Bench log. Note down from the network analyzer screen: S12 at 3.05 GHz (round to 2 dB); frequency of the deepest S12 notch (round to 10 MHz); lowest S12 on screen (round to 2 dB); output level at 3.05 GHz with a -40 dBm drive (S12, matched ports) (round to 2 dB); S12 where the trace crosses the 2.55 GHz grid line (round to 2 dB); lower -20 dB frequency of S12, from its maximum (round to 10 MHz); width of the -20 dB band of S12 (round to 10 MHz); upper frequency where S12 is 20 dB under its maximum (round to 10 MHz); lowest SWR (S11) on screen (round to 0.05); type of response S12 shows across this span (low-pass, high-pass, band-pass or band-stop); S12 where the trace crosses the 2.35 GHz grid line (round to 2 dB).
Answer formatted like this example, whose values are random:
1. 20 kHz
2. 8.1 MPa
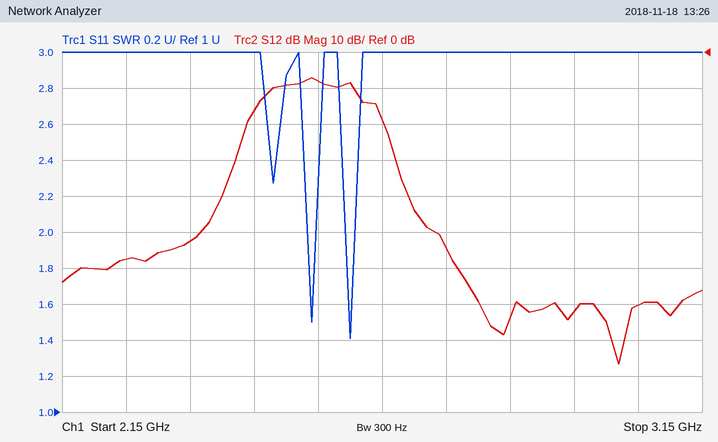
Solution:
1. -70 dB
2. 3.02 GHz
3. -86 dB
4. -110 dBm
5. -8 dB
6. 2.43 GHz
7. 240 MHz
8. 2.67 GHz
9. 1.40
10. band-pass
11. -52 dB
